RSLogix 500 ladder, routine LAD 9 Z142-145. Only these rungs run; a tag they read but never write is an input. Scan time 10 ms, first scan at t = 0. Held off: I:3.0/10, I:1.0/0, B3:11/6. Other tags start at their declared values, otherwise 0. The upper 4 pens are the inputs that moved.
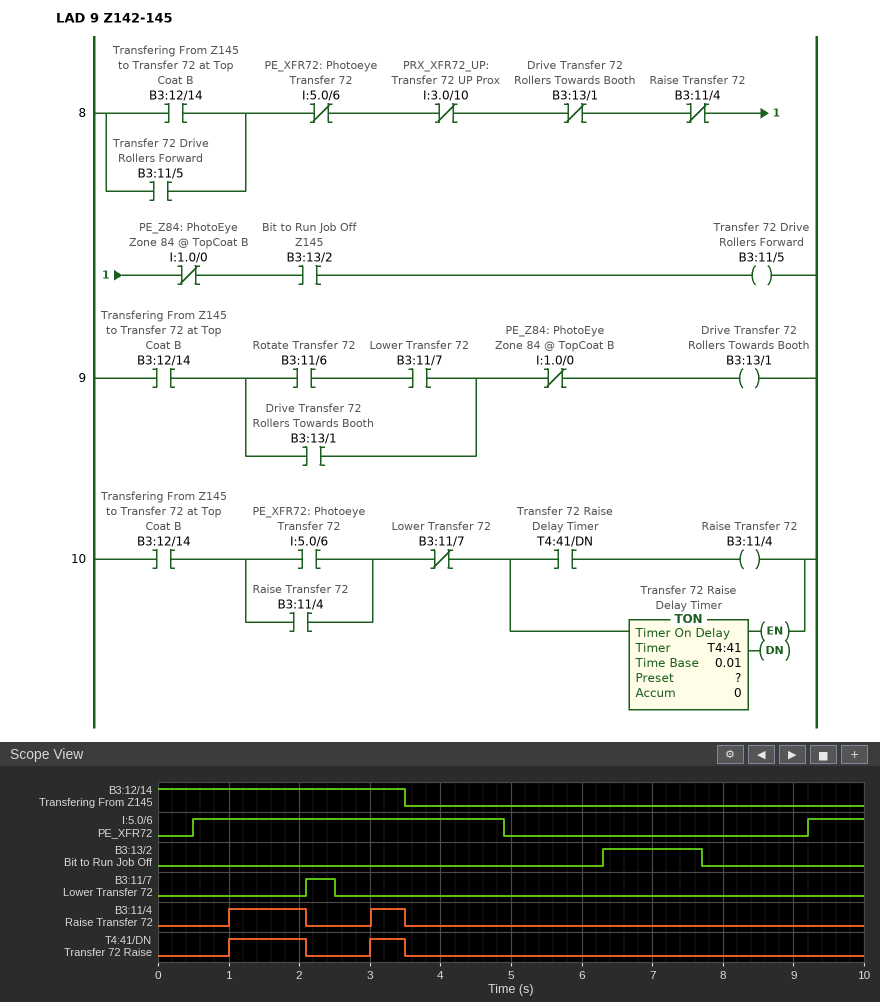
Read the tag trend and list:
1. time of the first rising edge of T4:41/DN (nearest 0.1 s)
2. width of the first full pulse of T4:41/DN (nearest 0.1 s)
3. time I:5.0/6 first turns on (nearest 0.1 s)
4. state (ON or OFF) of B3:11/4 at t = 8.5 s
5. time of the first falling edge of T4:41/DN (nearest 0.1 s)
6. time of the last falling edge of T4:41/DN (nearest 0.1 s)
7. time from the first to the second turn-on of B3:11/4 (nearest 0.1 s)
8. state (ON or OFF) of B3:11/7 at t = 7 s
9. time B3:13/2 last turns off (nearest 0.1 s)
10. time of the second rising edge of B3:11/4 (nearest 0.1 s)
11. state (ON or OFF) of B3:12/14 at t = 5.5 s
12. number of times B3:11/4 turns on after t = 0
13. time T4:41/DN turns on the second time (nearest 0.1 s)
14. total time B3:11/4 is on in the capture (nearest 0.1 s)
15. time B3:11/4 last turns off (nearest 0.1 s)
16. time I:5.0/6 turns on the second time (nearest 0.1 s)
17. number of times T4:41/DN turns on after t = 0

1.0 s
1.1 s
0.5 s
OFF
2.1 s
3.5 s
2.0 s
OFF
7.7 s
3.0 s
OFF
2
3.0 s
1.6 s
3.5 s
9.2 s
2
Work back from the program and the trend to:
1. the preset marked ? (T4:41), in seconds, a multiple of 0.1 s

0.5 s
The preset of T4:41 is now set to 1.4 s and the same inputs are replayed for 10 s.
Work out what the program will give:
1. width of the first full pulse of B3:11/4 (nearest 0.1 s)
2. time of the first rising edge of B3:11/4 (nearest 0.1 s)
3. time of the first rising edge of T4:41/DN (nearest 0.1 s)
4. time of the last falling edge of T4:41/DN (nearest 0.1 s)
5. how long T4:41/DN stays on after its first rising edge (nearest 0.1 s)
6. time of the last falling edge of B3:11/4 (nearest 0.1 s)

0.2 s
1.9 s
1.9 s
2.1 s
0.2 s
2.1 s
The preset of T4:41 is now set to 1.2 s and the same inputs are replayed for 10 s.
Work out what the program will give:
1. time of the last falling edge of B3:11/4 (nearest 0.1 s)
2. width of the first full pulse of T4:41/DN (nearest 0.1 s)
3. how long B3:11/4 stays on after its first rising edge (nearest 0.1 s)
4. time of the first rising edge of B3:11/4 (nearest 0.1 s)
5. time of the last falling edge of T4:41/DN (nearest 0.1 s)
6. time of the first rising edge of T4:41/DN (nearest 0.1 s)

2.1 s
0.4 s
0.4 s
1.7 s
2.1 s
1.7 s
